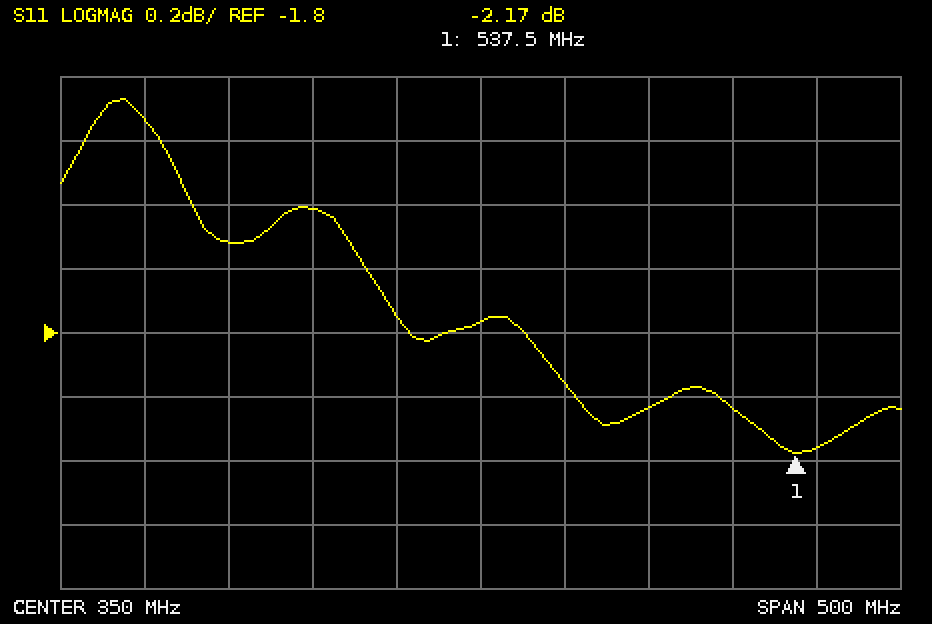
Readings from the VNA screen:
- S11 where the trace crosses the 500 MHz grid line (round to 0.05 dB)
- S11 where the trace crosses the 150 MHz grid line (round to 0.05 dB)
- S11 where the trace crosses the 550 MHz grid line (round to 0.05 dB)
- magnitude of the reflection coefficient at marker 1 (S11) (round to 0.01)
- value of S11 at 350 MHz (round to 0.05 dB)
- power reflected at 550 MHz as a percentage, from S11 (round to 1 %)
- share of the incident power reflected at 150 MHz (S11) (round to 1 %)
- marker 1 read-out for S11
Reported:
-2.05 dB
-1.15 dB
-2.15 dB
0.78
-1.75 dB
61 %
77 %
-2.17 dB
